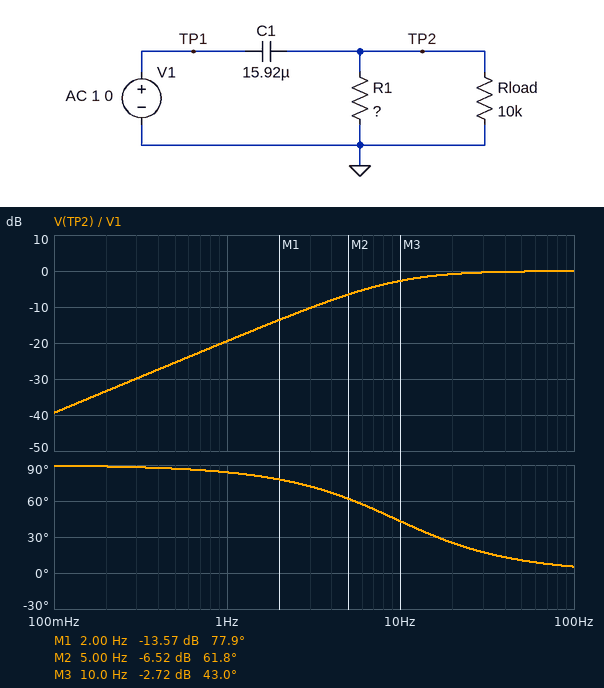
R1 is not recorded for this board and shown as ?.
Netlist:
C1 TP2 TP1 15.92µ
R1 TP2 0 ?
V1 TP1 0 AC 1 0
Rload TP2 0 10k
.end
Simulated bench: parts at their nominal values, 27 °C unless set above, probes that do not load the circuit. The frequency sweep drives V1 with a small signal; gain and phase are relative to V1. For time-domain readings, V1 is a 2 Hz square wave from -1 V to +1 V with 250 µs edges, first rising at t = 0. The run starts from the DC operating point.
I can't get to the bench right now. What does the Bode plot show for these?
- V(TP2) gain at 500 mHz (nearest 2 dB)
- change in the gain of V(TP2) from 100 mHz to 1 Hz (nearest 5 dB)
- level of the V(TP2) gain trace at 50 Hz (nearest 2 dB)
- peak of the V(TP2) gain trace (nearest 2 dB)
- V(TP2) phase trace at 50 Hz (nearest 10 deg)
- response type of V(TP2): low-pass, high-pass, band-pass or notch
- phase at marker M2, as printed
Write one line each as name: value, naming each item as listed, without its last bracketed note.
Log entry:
V(TP2) gain at 500 mHz: -26 dB
change in the gain of V(TP2) from 100 mHz to 1 Hz: 20 dB
level of the V(TP2) gain trace at 50 Hz: 0 dB
peak of the V(TP2) gain trace: 0 dB
V(TP2) phase trace at 50 Hz: 10 deg
response type of V(TP2): low-pass, high-pass, band-pass or notch: high-pass
phase at marker M2, as printed: 61.8 deg
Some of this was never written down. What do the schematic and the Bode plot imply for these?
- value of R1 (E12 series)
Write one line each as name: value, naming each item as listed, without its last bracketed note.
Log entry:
value of R1: 1.2 kΩ
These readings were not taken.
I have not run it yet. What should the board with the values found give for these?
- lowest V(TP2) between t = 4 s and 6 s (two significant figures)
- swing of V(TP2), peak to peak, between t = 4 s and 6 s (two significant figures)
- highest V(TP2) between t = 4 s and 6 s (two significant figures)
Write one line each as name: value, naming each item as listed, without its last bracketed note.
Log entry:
lowest V(TP2) between t = 4 s and 6 s: -2.0 V
swing of V(TP2), peak to peak, between t = 4 s and 6 s: 4.0 V
highest V(TP2) between t = 4 s and 6 s: 2.0 V
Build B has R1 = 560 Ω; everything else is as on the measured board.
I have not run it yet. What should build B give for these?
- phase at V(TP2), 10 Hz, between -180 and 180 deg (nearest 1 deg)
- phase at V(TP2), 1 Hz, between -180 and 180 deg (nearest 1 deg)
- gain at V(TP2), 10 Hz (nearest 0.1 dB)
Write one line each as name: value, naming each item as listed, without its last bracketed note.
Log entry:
phase at V(TP2), 10 Hz, between -180 and 180 deg: 62 deg
phase at V(TP2), 1 Hz, between -180 and 180 deg: 87 deg
gain at V(TP2), 10 Hz: -6.6 dB
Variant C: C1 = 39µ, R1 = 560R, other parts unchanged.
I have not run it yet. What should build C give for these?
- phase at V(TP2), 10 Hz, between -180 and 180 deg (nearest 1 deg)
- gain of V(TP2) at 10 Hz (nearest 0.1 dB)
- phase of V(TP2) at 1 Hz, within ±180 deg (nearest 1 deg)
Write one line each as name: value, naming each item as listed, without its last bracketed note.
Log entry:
phase at V(TP2), 10 Hz, between -180 and 180 deg: 38 deg
gain of V(TP2) at 10 Hz: -2.0 dB
phase of V(TP2) at 1 Hz, within ±180 deg: 83 deg
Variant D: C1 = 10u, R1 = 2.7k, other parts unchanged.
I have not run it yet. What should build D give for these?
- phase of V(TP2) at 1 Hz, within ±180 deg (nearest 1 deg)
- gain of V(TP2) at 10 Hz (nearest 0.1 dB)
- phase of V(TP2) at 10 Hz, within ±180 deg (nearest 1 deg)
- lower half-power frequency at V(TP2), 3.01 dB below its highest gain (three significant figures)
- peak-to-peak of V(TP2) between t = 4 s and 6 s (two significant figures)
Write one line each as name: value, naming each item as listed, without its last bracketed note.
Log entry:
phase of V(TP2) at 1 Hz, within ±180 deg: 82 deg
gain of V(TP2) at 10 Hz: -1.9 dB
phase of V(TP2) at 10 Hz, within ±180 deg: 37 deg
lower half-power frequency at V(TP2), 3.01 dB below its highest gain: 7.49 Hz
peak-to-peak of V(TP2) between t = 4 s and 6 s: 4.0 V
